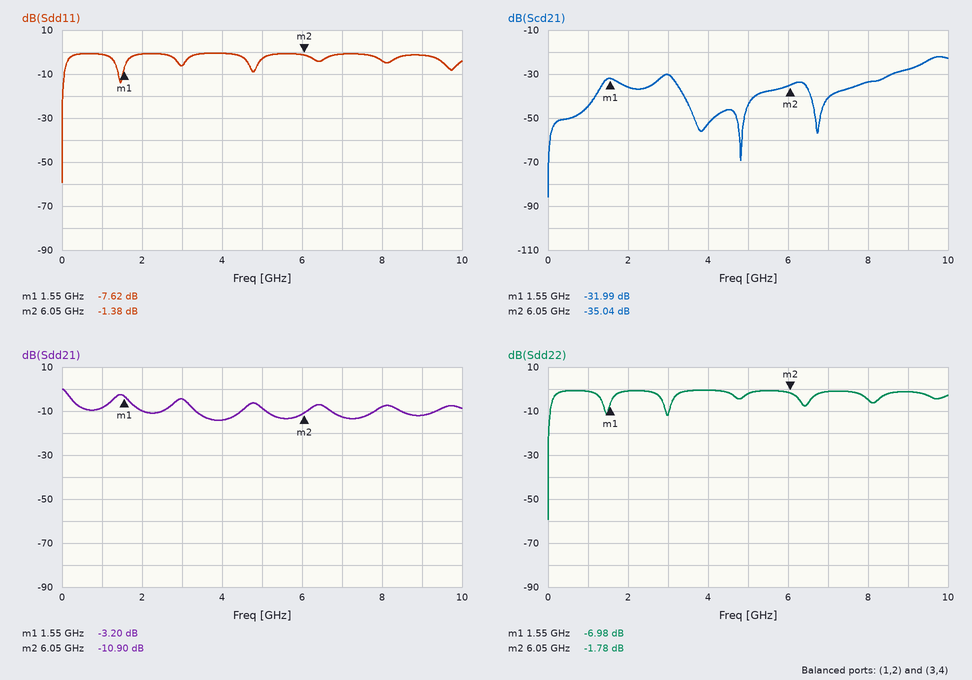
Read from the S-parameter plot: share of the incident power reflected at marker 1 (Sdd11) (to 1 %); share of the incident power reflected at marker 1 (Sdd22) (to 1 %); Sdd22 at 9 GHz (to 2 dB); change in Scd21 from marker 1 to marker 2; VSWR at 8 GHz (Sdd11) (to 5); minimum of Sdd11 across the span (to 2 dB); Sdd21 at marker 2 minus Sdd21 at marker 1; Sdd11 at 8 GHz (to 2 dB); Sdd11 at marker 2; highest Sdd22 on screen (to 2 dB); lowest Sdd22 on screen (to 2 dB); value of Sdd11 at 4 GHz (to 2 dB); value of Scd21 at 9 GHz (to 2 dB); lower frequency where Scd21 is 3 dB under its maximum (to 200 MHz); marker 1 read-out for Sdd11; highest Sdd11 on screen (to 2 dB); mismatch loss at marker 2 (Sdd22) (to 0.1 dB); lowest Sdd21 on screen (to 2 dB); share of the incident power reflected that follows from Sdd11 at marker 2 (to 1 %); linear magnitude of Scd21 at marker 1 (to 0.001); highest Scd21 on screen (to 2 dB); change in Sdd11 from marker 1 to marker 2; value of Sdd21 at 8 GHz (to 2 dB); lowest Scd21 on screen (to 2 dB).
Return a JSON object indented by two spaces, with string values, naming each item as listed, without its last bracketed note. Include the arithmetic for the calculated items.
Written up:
{
  "share of the incident power reflected at marker 1 (Sdd11)": "10^(-7.62/10) ≈ 17 %",
  "share of the incident power reflected at marker 1 (Sdd22)": "10^(-6.98/10) ≈ 20 %",
  "Sdd22 at 9 GHz": "-2 dB",
  "change in Scd21 from marker 1 to marker 2": "-35.04 − (-31.99) = -3.05 dB",
  "VSWR at 8 GHz (Sdd11)": "|Γ| = 10^(-4/20) = 0.6310; VSWR = (1 + 0.6310)/(1 − 0.6310) ≈ 4.42, so 5 to the nearest 5",
  "minimum of Sdd11 across the span": "-60 dB",
  "Sdd21 at marker 2 minus Sdd21 at marker 1": "-10.9 − (-3.2) = -7.70 dB",
  "Sdd11 at 8 GHz": "-4 dB",
  "Sdd11 at marker 2": "-1.38 dB",
  "highest Sdd22 on screen": "0 dB",
  "lowest Sdd22 on screen": "-60 dB",
  "value of Sdd11 at 4 GHz": "0 dB",
  "value of Scd21 at 9 GHz": "-28 dB",
  "lower frequency where Scd21 is 3 dB under its maximum": "9.4 GHz",
  "marker 1 read-out for Sdd11": "-7.62 dB",
  "highest Sdd11 on screen": "0 dB",
  "mismatch loss at marker 2 (Sdd22)": "−10 log10(1 − 10^(-1.78/10)) ≈ 4.7 dB",
  "lowest Sdd21 on screen": "-14 dB",
  "share of the incident power reflected that follows from Sdd11 at marker 2": "10^(-1.38/10) ≈ 73 %",
  "linear magnitude of Scd21 at marker 1": "10^(-31.99/20) ≈ 0.025",
  "highest Scd21 on screen": "-22 dB",
  "change in Sdd11 from marker 1 to marker 2": "-1.38 − (-7.62) = 6.24 dB",
  "value of Sdd21 at 8 GHz": "-8 dB",
  "lowest Scd21 on screen": "-86 dB"
}
